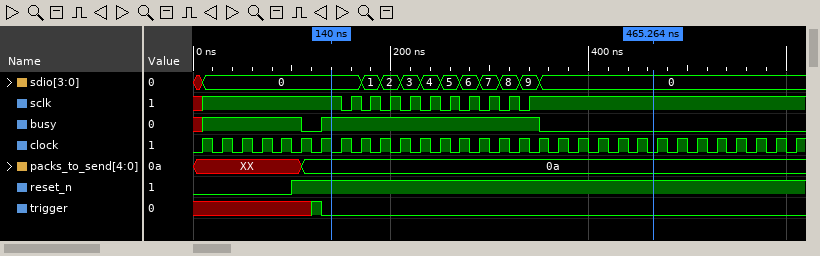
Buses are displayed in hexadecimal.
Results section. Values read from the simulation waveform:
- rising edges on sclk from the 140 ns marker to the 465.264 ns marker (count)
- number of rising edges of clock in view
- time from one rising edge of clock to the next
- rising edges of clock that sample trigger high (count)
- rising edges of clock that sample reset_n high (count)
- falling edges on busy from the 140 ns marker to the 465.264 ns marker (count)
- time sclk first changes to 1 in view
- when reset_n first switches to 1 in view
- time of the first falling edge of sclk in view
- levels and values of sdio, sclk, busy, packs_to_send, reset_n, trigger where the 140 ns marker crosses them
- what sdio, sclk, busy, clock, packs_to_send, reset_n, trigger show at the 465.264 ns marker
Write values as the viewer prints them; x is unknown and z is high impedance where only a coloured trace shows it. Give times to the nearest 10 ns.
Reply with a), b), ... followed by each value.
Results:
a) 10
b) 31
c) 20 ns
d) 1
e) 26
f) 1
g) 10 ns
h) 100 ns
i) 150 ns
j) sdio=0, sclk=1, busy=1, packs_to_send=0a, reset_n=1, trigger=0
k) sdio=0, sclk=1, busy=0, clock=0, packs_to_send=0a, reset_n=1, trigger=0
